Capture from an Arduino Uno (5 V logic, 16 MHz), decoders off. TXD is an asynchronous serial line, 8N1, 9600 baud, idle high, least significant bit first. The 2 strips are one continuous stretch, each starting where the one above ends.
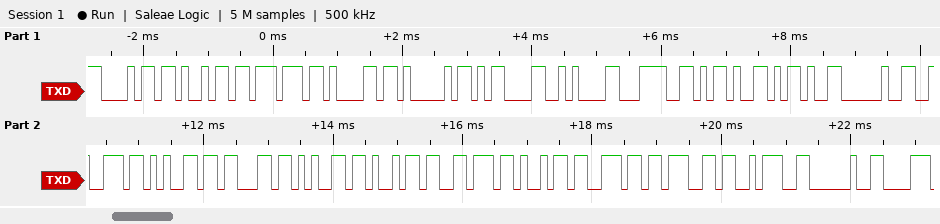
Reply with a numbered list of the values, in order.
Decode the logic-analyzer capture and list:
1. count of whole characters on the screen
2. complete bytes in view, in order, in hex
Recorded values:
1. 22
2. 0x68 0x69 0x77 0x61 0x41 0x0D 0x0A 0x3C 0x2D 0x2D 0x20 0x72 0x65 0x63 0x65 0x69 0x76 0x69 0x6E 0x67 0x3A 0x20
